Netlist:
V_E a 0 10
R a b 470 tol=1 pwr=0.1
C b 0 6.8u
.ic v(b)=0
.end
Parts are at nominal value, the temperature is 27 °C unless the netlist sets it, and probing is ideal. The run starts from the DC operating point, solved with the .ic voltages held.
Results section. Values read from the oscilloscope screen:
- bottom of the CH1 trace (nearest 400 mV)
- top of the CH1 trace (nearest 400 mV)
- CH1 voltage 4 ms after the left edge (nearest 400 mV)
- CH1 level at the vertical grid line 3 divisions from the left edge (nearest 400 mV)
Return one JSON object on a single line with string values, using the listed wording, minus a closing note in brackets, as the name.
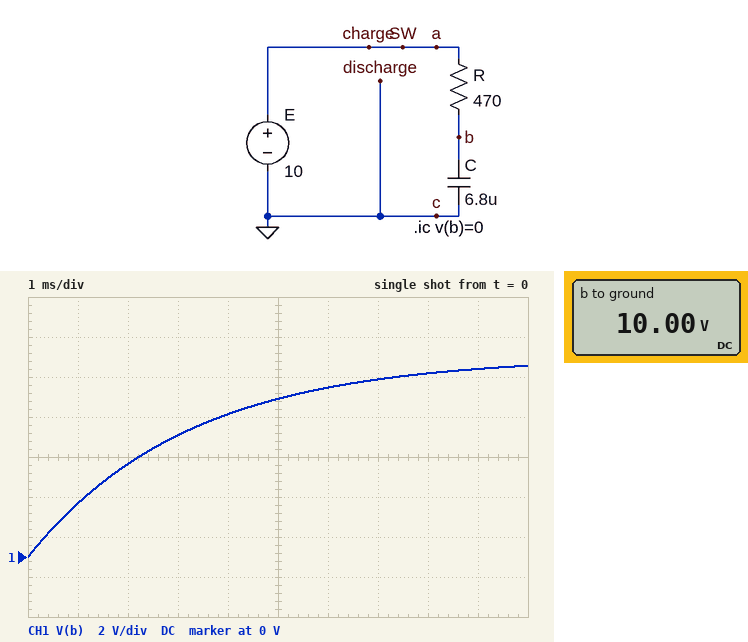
{"bottom of the CH1 trace": "0 V", "top of the CH1 trace": "9.6 V", "CH1 voltage 4 ms after the left edge": "7.2 V", "CH1 level at the vertical grid line 3 divisions from the left edge": "6.0 V"}
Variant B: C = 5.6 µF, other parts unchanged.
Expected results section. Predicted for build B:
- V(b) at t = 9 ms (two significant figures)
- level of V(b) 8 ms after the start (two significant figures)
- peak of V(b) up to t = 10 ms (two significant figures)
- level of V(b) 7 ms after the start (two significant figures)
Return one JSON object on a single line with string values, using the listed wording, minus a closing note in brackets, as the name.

{"V(b) at t = 9 ms": "9.7 V", "level of V(b) 8 ms after the start": "9.5 V", "peak of V(b) up to t = 10 ms": "9.8 V", "level of V(b) 7 ms after the start": "9.3 V"}
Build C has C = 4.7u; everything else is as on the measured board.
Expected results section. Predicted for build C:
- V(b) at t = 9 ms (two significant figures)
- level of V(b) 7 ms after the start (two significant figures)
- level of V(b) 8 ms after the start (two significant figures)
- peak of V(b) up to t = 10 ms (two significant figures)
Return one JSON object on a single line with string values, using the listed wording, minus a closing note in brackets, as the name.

{"V(b) at t = 9 ms": "9.8 V", "level of V(b) 7 ms after the start": "9.6 V", "level of V(b) 8 ms after the start": "9.7 V", "peak of V(b) up to t = 10 ms": "9.9 V"}
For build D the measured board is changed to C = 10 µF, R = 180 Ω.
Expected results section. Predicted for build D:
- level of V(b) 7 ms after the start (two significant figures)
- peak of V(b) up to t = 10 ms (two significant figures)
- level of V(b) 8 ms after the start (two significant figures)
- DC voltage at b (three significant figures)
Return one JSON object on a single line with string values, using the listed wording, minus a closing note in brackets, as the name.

{"level of V(b) 7 ms after the start": "9.8 V", "peak of V(b) up to t = 10 ms": "10 V", "level of V(b) 8 ms after the start": "9.9 V", "DC voltage at b": "10.0 V"}
